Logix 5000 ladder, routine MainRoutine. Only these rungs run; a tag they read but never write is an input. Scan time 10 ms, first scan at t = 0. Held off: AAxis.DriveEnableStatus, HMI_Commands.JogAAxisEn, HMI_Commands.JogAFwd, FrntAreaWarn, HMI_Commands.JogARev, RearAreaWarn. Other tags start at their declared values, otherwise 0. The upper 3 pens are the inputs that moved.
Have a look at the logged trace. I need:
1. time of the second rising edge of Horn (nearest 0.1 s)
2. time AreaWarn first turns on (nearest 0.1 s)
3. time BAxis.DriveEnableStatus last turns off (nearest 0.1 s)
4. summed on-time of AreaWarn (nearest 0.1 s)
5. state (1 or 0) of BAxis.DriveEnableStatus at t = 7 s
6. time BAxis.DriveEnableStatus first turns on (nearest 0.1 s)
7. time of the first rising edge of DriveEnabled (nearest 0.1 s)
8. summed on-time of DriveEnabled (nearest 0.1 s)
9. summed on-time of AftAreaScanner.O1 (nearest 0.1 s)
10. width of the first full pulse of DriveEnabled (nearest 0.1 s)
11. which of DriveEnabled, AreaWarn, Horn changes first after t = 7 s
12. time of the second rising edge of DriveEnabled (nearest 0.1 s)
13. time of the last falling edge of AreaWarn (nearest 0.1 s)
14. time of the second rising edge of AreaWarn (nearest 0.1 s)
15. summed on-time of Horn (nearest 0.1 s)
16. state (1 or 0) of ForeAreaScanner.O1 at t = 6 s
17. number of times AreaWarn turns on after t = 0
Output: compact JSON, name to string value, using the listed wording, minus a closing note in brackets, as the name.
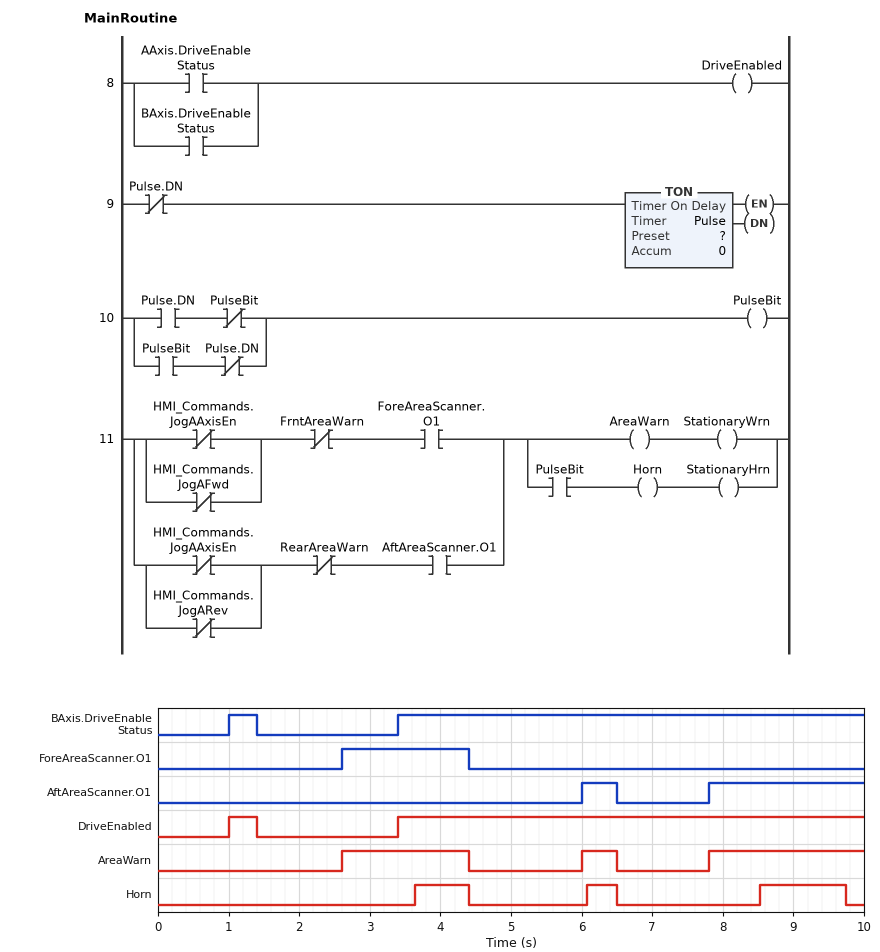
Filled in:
{"time of the second rising edge of Horn": "6.1 s", "time AreaWarn first turns on": "2.6 s", "time BAxis.DriveEnableStatus last turns off": "1.4 s", "summed on-time of AreaWarn": "4.5 s", "state (1 or 0) of BAxis.DriveEnableStatus at t = 7 s": "1", "time BAxis.DriveEnableStatus first turns on": "1.0 s", "time of the first rising edge of DriveEnabled": "1.0 s", "summed on-time of DriveEnabled": "7.0 s", "summed on-time of AftAreaScanner.O1": "2.7 s", "width of the first full pulse of DriveEnabled": "0.4 s", "which of DriveEnabled, AreaWarn, Horn changes first after t = 7 s": "AreaWarn", "time of the second rising edge of DriveEnabled": "3.4 s", "time of the last falling edge of AreaWarn": "6.5 s", "time of the second rising edge of AreaWarn": "6.0 s", "summed on-time of Horn": "2.4 s", "state (1 or 0) of ForeAreaScanner.O1 at t = 6 s": "0", "number of times AreaWarn turns on after t = 0": "3"}
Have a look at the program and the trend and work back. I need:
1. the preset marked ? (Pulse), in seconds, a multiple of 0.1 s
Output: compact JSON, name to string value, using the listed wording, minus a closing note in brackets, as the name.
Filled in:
{"the preset marked ? (Pulse), in seconds, a multiple of 0.1 s": "1.2 s"}
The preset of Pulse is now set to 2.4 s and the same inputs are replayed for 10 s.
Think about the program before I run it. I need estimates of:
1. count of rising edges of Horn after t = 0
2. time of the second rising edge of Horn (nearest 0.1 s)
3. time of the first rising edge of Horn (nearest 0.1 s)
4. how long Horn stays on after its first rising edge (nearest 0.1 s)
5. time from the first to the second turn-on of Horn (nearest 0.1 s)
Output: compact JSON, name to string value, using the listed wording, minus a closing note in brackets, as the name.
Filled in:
{"count of rising edges of Horn after t = 0": "2", "time of the second rising edge of Horn": "7.8 s", "time of the first rising edge of Horn": "2.6 s", "how long Horn stays on after its first rising edge": "1.8 s", "time from the first to the second turn-on of Horn": "5.2 s"}
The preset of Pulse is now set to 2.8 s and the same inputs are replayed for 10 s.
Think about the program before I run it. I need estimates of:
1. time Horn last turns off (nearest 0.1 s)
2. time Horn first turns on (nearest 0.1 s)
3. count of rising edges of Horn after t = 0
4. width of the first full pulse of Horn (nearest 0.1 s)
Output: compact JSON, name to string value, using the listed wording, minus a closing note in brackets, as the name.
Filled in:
{"time Horn last turns off": "4.4 s", "time Horn first turns on": "2.8 s", "count of rising edges of Horn after t = 0": "2", "width of the first full pulse of Horn": "1.6 s"}
